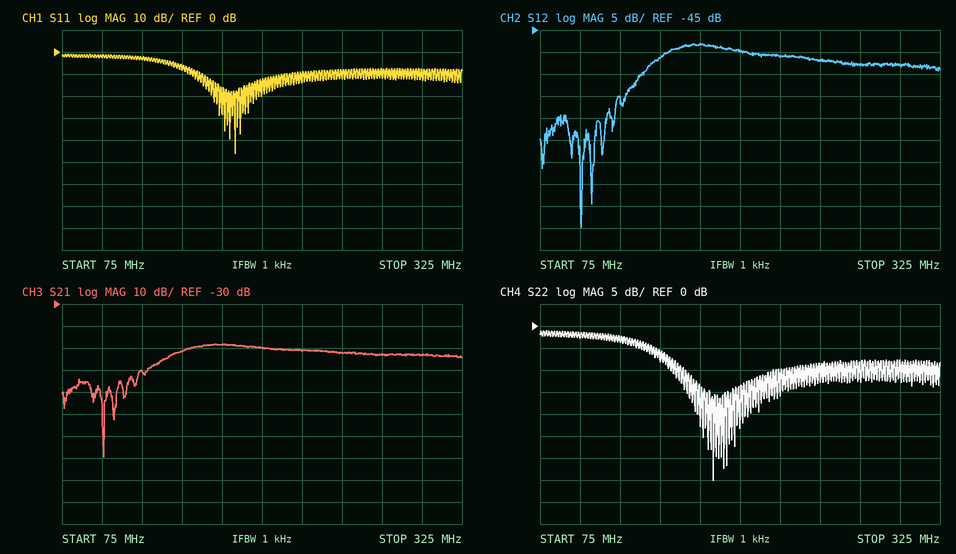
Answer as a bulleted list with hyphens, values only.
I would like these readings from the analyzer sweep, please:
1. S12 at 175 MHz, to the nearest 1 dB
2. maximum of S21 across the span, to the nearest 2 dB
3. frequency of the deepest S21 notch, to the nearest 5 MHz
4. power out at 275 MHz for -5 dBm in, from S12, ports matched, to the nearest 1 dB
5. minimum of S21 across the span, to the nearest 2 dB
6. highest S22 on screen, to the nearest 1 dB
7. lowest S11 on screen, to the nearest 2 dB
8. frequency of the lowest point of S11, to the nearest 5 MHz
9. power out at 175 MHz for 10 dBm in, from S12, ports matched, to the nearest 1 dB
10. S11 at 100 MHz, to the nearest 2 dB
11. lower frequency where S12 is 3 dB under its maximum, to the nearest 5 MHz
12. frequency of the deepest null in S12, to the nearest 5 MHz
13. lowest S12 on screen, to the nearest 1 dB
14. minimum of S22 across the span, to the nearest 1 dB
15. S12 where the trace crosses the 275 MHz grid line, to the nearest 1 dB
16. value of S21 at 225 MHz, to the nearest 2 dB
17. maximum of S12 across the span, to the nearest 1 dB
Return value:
- -48 dB
- -48 dB
- 100 MHz
- -58 dBm
- -100 dB
- -1 dB
- -46 dB
- 185 MHz
- -38 dBm
- -2 dB
- 150 MHz
- 100 MHz
- -90 dB
- -35 dB
- -53 dB
- -52 dB
- -48 dB
